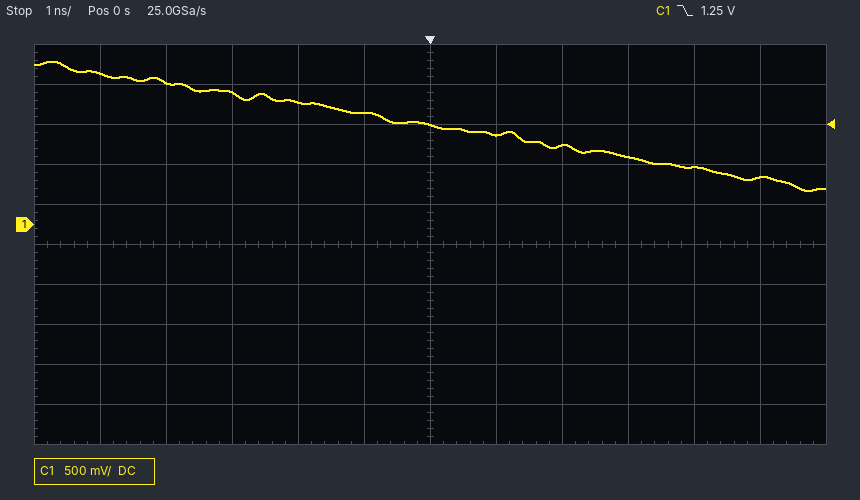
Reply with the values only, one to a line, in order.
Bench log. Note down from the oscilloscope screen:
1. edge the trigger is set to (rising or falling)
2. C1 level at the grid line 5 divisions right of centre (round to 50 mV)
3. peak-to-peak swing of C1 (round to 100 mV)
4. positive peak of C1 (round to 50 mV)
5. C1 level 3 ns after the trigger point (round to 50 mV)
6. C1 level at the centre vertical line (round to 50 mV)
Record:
falling
600 mV
1.60 V
2.05 V
850 mV
1.25 V
